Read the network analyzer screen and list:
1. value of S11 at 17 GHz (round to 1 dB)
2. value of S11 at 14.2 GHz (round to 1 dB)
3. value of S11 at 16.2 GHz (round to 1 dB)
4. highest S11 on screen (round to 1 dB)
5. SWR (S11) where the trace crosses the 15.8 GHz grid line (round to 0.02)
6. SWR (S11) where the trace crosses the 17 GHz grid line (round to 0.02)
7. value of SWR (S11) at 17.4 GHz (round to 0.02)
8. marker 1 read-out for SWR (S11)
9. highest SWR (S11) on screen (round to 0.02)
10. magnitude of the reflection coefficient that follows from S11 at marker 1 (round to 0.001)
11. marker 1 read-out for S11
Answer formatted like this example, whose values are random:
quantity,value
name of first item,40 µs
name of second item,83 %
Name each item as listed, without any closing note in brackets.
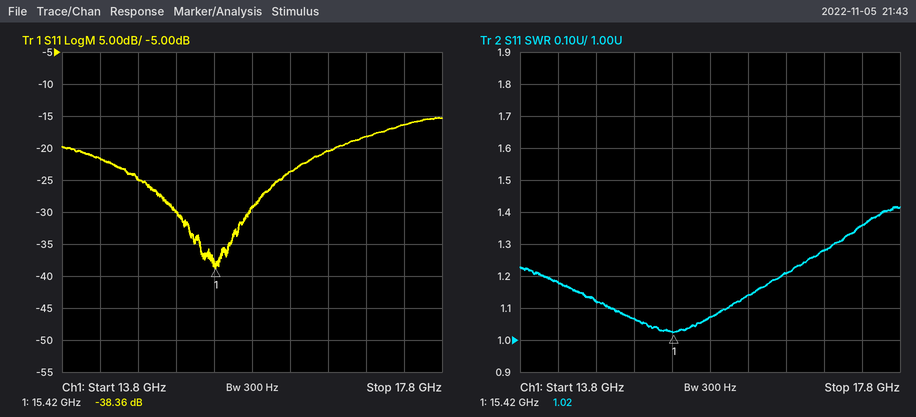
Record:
quantity,value
value of S11 at 17 GHz,-18 dB
value of S11 at 14.2 GHz,-22 dB
value of S11 at 16.2 GHz,-24 dB
highest S11 on screen,-15 dB
SWR (S11) where the trace crosses the 15.8 GHz grid line,1.08
SWR (S11) where the trace crosses the 17 GHz grid line,1.28
value of SWR (S11) at 17.4 GHz,1.36
marker 1 read-out for SWR,1.02
highest SWR (S11) on screen,1.42
magnitude of the reflection coefficient that follows from S11 at marker 1,0.012
marker 1 read-out for S11,-38.36 dB
